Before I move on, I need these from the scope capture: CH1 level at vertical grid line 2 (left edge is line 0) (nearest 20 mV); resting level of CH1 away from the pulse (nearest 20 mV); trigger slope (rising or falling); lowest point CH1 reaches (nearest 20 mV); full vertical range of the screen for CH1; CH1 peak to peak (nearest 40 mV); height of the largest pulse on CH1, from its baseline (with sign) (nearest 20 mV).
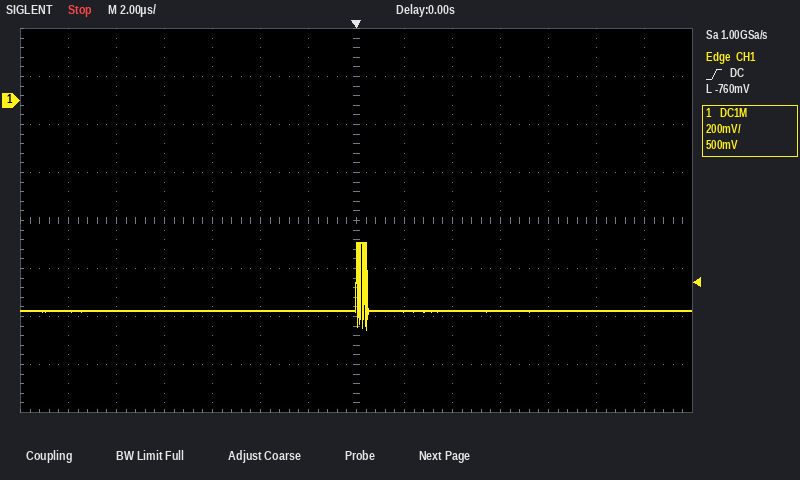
-880 mV
-880 mV
rising
-960 mV
1.6 V
360 mV
+280 mV
